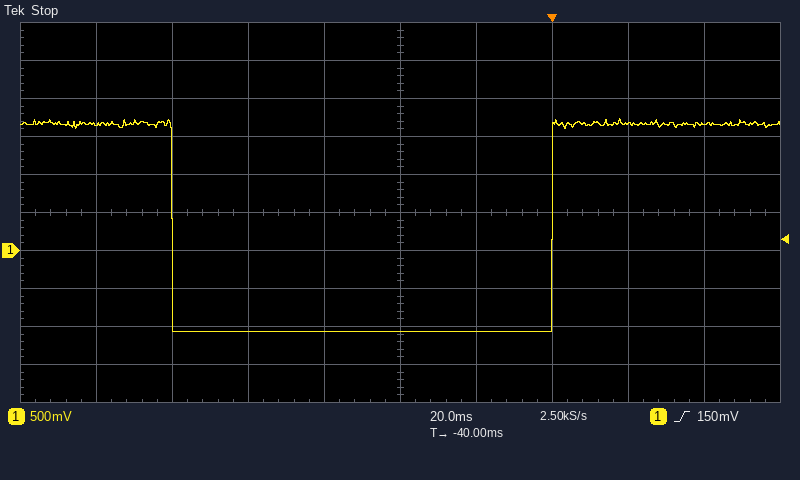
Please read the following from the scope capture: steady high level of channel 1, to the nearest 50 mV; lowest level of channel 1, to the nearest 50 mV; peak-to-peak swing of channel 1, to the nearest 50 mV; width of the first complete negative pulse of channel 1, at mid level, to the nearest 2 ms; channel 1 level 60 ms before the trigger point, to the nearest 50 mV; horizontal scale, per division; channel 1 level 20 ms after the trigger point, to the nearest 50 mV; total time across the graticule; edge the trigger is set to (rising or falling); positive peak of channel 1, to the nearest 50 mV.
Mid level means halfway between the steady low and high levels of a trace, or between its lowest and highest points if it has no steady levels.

1.65 V
-1.05 V
2.80 V
100 ms
-1.05 V
20 ms
1.65 V
200 ms
rising
1.75 V
